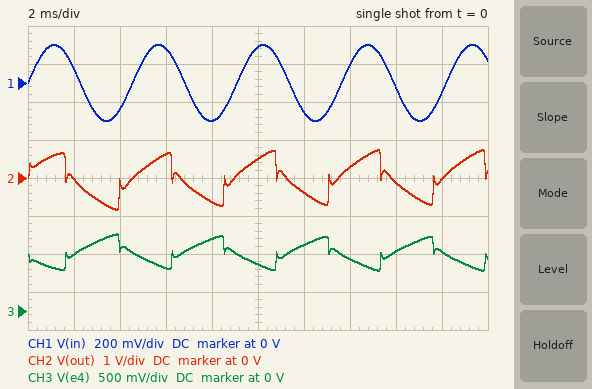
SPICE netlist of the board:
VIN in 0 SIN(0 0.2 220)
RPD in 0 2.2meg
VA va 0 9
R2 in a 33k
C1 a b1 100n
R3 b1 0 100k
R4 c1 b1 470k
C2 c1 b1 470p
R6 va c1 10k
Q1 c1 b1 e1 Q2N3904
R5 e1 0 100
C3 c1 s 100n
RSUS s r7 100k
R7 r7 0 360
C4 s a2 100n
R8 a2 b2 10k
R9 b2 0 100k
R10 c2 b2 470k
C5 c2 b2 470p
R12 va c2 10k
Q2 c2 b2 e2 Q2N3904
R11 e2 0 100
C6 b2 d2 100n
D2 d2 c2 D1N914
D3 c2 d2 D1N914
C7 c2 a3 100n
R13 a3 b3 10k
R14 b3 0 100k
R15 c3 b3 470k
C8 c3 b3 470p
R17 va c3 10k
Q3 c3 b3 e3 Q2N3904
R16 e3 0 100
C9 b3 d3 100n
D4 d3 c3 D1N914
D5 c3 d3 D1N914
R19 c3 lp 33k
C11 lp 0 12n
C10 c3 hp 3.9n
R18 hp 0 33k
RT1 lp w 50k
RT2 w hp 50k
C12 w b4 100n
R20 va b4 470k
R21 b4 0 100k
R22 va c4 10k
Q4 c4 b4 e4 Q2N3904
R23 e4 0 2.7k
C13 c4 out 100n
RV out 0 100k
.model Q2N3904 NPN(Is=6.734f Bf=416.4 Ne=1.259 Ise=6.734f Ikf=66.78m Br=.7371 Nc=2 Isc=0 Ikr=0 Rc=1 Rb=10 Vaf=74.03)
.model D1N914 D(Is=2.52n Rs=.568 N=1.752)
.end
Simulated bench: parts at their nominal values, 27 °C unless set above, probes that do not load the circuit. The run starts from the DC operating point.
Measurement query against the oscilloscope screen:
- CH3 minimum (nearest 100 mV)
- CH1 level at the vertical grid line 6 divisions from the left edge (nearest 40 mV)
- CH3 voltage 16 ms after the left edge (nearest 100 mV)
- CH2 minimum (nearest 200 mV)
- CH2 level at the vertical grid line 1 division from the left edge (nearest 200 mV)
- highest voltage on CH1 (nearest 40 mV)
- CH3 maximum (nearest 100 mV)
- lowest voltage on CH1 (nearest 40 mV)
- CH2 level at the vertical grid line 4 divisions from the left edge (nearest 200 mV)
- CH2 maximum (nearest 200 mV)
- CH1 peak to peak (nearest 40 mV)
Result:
500 mV
-160 mV
800 mV
-800 mV
0 V
200 mV
1.0 V
-200 mV
-600 mV
800 mV
400 mV
